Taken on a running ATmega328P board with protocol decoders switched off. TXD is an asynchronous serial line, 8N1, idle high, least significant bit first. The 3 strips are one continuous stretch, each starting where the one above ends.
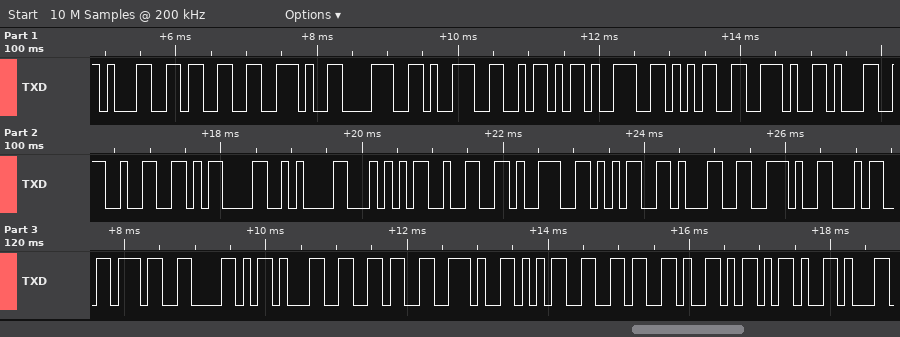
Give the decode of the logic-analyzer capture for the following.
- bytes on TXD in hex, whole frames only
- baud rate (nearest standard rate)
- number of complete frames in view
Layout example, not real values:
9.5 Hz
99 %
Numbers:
31 33 2E 38 39 5A 39 35 2E 31 32 0D 0A 54 32 39 35 31 2E 34 37 58 31 36 2E 35 36 59 2D
9600 baud
29
